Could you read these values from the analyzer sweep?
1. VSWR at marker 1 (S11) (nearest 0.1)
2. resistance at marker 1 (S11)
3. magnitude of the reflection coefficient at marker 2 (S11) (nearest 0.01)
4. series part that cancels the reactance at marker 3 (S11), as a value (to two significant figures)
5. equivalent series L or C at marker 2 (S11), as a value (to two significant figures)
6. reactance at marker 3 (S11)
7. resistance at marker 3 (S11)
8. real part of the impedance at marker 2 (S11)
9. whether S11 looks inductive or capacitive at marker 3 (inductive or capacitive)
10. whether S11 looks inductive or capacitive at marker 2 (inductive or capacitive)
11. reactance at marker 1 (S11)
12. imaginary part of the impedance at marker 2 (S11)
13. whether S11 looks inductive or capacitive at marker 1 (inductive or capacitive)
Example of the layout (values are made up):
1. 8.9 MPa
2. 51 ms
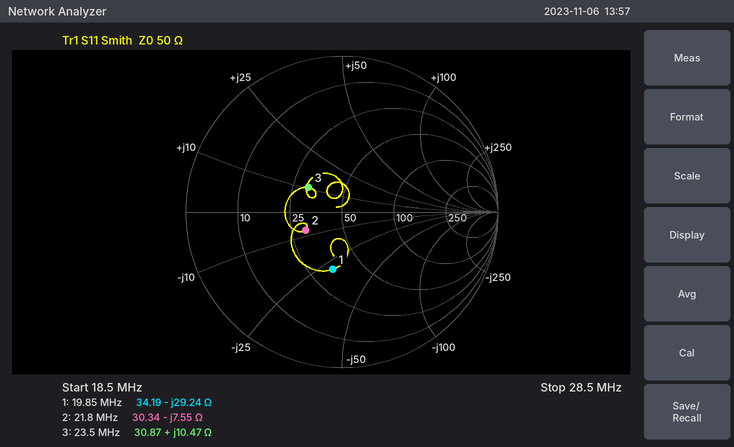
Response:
1. 2.2
2. 34.19 Ω
3. 0.26
4. 650 pF
5. 970 pF
6. +10.47 Ω
7. 30.87 Ω
8. 30.34 Ω
9. inductive
10. capacitive
11. -29.24 Ω
12. -7.55 Ω
13. capacitive
